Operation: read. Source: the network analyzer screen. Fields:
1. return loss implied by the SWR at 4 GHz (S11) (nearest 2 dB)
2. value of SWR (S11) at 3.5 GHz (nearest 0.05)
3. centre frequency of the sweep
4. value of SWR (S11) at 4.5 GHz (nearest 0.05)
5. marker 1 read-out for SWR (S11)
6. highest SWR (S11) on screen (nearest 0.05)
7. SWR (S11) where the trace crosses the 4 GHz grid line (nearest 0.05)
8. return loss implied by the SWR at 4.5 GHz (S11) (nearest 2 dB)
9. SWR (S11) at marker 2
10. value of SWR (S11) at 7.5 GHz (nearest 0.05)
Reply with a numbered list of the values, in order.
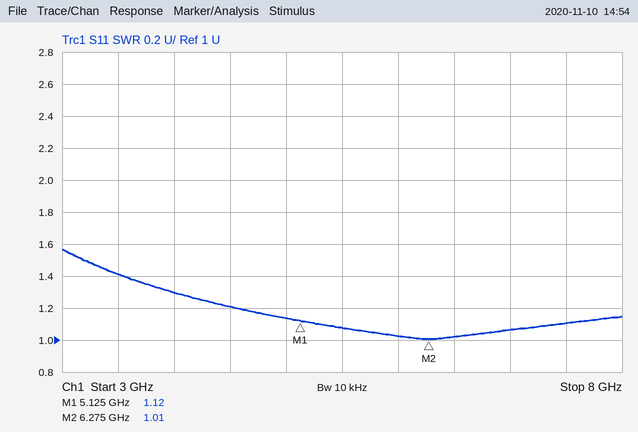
1. 18 dB
2. 1.40
3. 5.5 GHz
4. 1.20
5. 1.12
6. 1.55
7. 1.30
8. 20 dB
9. 1.01
10. 1.10
